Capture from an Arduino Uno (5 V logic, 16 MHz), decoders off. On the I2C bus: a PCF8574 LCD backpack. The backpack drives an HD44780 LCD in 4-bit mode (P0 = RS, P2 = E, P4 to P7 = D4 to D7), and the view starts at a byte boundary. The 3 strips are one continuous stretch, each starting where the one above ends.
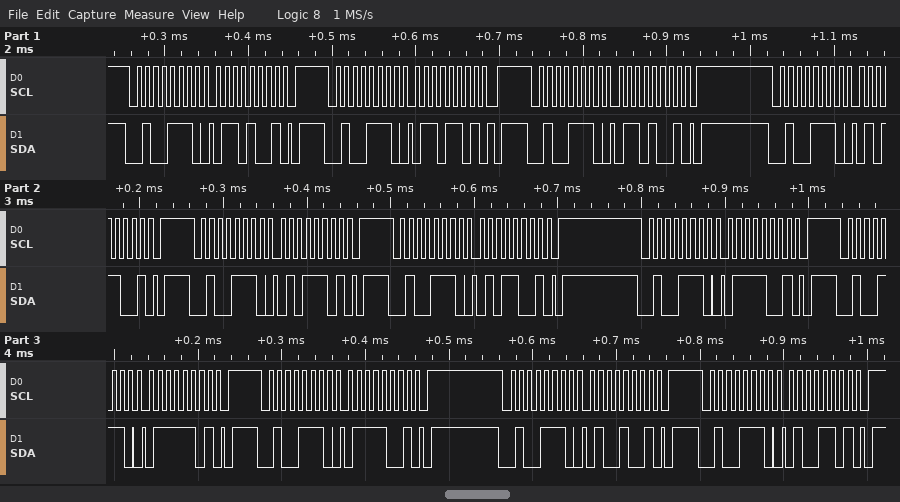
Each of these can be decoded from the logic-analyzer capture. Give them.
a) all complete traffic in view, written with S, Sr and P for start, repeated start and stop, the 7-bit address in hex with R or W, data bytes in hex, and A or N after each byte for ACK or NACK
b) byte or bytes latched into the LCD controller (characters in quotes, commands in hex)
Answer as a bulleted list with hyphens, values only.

- S 27W A 69 A P S 27W A 6D A P S 27W A 69 A P S 27W A 59 A P S 27W A 5D A P S 27W A 59 A P S 27W A 79 A P S 27W A 7D A P S 27W A 79 A P S 27W A 49 A P S 27W A 4D A P
- 'e'
